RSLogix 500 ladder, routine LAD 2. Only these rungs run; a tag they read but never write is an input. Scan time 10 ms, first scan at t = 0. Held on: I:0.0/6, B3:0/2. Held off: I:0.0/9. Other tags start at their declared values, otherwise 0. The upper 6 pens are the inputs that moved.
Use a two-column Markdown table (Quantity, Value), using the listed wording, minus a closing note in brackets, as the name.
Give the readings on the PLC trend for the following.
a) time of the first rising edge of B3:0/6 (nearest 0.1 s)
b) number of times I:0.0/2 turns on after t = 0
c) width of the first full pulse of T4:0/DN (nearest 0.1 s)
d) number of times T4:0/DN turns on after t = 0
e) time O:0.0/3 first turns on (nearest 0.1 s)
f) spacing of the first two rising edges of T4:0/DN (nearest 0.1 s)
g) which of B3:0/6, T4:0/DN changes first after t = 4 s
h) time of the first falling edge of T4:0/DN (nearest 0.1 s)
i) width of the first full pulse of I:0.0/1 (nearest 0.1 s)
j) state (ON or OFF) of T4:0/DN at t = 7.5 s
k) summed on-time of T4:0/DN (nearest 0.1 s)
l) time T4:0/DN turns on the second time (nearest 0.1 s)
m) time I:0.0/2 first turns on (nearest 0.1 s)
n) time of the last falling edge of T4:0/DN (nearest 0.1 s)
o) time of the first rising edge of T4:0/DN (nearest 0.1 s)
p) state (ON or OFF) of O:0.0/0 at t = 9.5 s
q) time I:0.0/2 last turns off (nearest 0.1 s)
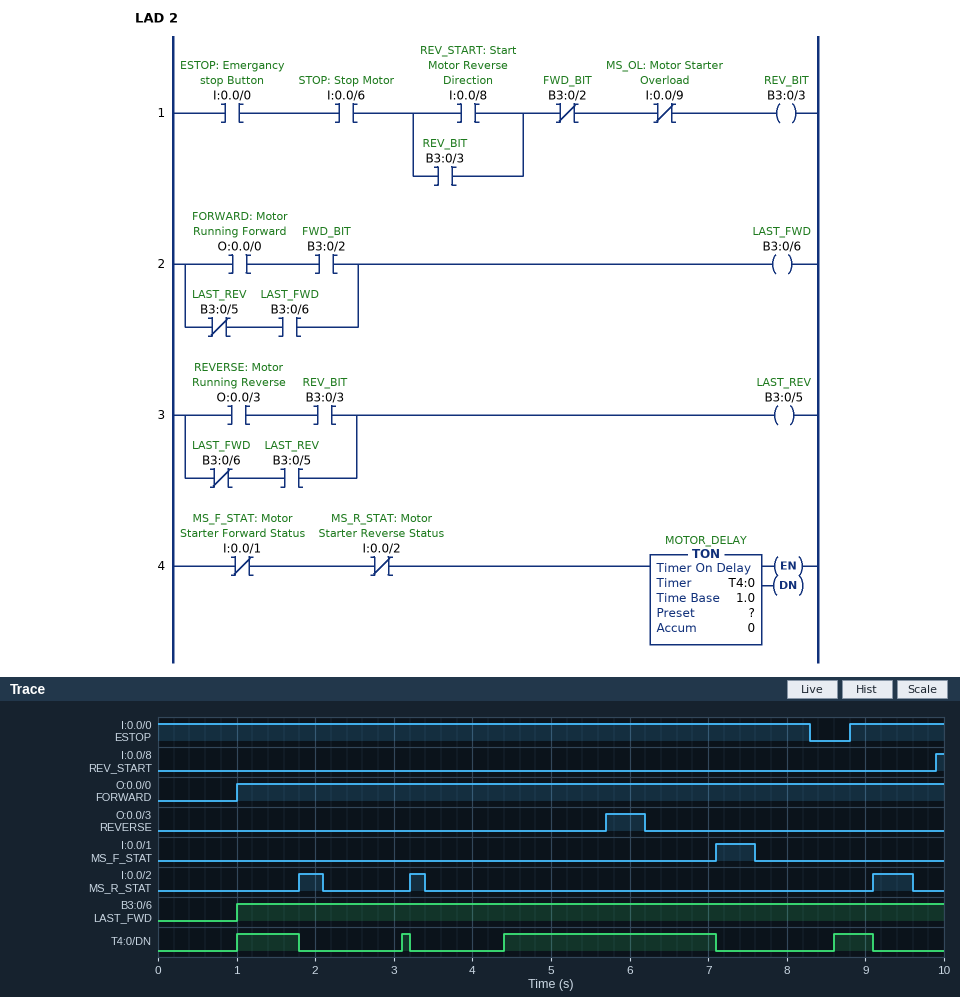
| Quantity | Value |
|---|---|
| time of the first rising edge of B3:0/6 | 1.0 s |
| number of times I:0.0/2 turns on after t = 0 | 3 |
| width of the first full pulse of T4:0/DN | 0.8 s |
| number of times T4:0/DN turns on after t = 0 | 4 |
| time O:0.0/3 first turns on | 5.7 s |
| spacing of the first two rising edges of T4:0/DN | 2.1 s |
| which of B3:0/6, T4:0/DN changes first after t = 4 s | T4:0/DN |
| time of the first falling edge of T4:0/DN | 1.8 s |
| width of the first full pulse of I:0.0/1 | 0.5 s |
| state (ON or OFF) of T4:0/DN at t = 7.5 s | OFF |
| summed on-time of T4:0/DN | 4.1 s |
| time T4:0/DN turns on the second time | 3.1 s |
| time I:0.0/2 first turns on | 1.8 s |
| time of the last falling edge of T4:0/DN | 9.1 s |
| time of the first rising edge of T4:0/DN | 1.0 s |
| state (ON or OFF) of O:0.0/0 at t = 9.5 s | ON |
| time I:0.0/2 last turns off | 9.6 s |
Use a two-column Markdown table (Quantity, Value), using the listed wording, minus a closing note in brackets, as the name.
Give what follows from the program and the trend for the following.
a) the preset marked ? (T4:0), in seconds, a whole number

| Quantity | Value |
|---|---|
| the preset marked ? (T4:0), in seconds, a whole number | 1 s |
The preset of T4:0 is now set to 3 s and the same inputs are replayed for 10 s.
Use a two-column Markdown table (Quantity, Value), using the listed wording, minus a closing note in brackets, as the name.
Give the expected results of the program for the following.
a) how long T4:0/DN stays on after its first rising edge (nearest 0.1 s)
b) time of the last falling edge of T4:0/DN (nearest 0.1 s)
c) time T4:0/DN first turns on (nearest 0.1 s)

| Quantity | Value |
|---|---|
| how long T4:0/DN stays on after its first rising edge | 0.7 s |
| time of the last falling edge of T4:0/DN | 7.1 s |
| time T4:0/DN first turns on | 6.4 s |
